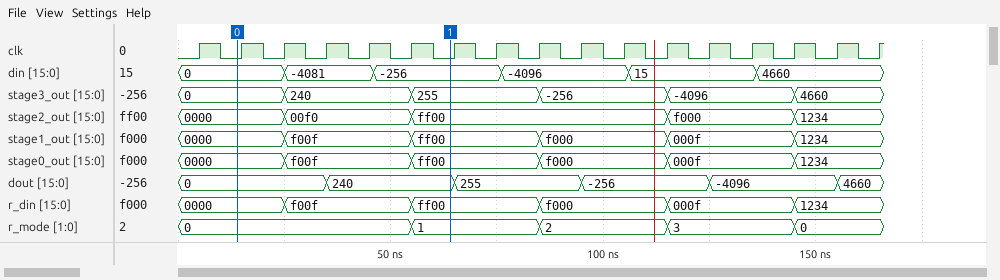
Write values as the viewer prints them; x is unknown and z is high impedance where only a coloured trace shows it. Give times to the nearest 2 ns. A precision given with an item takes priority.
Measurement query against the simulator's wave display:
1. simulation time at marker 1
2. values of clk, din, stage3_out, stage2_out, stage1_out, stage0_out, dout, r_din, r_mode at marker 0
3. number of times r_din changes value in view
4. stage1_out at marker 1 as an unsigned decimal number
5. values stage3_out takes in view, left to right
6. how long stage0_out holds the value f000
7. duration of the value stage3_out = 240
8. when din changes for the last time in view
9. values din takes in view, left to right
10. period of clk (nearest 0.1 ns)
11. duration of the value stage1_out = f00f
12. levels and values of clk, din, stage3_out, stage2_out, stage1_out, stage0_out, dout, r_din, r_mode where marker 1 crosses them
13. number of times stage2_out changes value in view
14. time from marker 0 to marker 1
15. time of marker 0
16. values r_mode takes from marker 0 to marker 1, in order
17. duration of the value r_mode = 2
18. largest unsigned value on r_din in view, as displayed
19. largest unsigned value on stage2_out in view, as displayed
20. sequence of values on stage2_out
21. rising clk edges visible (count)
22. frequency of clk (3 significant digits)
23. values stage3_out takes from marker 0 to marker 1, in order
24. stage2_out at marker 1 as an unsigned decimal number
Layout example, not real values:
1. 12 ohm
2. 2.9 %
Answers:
1. 64 ns
2. clk=0, din=0, stage3_out=0, stage2_out=0000, stage1_out=0000, stage0_out=0000, dout=0, r_din=0000, r_mode=0
3. 5
4. 65280
5. 0, 240, 255, -256, -4096, 4660
6. 30 ns
7. 30 ns
8. 136 ns
9. 0, -4081, -256, -4096, 15, 4660
10. 10 ns
11. 30 ns
12. clk=0, din=-256, stage3_out=255, stage2_out=ff00, stage1_out=ff00, stage0_out=ff00, dout=240, r_din=ff00, r_mode=1
13. 4
14. 50 ns
15. 14 ns
16. 0, 1
17. 30 ns
18. ff00
19. ff00
20. 0000, 00f0, ff00, f000, 1234
21. 17
22. 100 MHz
23. 0, 240, 255
24. 65280
